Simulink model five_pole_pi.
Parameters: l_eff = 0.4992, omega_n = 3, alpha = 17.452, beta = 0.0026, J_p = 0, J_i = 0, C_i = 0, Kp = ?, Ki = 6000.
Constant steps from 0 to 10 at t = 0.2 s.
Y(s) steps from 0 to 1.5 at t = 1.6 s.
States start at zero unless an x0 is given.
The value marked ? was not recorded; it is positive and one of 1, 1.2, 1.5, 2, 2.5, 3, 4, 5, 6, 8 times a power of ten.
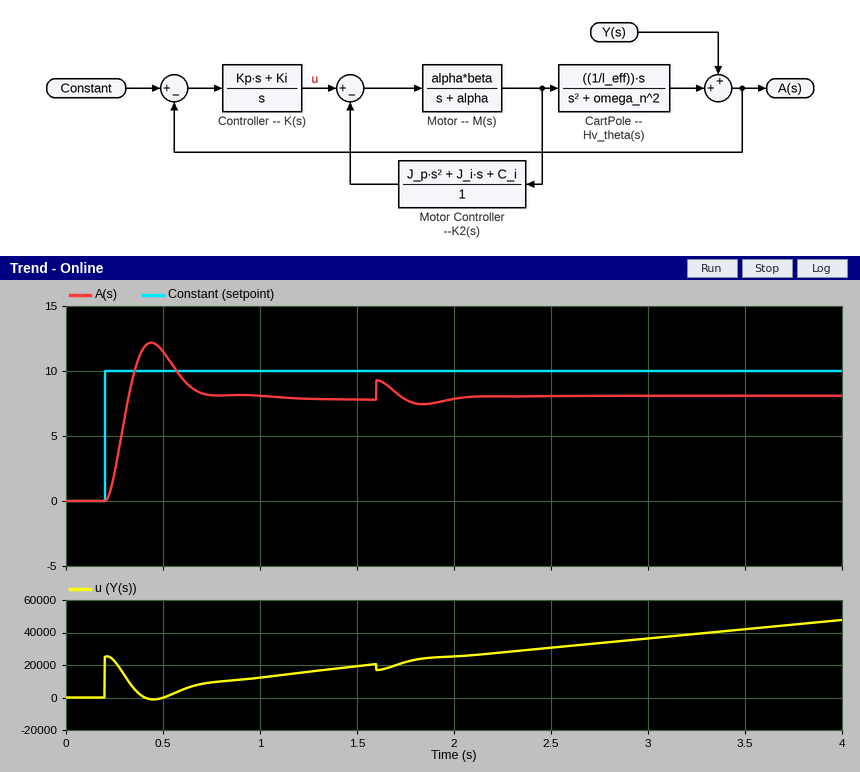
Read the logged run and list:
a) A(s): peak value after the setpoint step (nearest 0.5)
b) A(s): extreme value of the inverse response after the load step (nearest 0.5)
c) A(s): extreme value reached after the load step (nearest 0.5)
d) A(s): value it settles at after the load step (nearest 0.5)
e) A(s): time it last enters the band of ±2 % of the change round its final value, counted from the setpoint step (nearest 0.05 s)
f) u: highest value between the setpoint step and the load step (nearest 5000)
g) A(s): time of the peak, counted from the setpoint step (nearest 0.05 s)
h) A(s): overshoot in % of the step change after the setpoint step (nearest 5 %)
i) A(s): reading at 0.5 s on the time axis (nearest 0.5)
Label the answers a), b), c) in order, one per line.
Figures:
a) 12.0
b) 7.5
c) 9.5
d) 8.0
e) 0.95 s
f) 25000
g) 0.25 s
h) 55 %
i) 11.5
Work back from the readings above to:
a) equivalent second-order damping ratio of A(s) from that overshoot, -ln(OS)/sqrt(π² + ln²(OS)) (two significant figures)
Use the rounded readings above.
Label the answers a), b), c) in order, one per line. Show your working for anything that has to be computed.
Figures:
a) ln(0.55) = -0.598; 0.598 / sqrt(9.870 + 0.357) = 0.19
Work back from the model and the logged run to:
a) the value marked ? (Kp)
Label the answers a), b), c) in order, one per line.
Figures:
a) 2500
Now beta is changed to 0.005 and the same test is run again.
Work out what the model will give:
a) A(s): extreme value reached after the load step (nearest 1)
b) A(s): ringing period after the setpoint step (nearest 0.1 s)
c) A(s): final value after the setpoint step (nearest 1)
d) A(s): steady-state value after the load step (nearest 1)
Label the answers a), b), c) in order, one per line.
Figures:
a) 10
b) 0.3 s
c) 9
d) 9
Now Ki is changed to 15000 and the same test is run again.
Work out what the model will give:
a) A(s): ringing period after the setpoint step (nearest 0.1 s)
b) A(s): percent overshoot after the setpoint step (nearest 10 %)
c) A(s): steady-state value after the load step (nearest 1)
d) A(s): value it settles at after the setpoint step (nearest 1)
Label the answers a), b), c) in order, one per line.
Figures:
a) 0.5 s
b) 60 %
c) 9
d) 9
